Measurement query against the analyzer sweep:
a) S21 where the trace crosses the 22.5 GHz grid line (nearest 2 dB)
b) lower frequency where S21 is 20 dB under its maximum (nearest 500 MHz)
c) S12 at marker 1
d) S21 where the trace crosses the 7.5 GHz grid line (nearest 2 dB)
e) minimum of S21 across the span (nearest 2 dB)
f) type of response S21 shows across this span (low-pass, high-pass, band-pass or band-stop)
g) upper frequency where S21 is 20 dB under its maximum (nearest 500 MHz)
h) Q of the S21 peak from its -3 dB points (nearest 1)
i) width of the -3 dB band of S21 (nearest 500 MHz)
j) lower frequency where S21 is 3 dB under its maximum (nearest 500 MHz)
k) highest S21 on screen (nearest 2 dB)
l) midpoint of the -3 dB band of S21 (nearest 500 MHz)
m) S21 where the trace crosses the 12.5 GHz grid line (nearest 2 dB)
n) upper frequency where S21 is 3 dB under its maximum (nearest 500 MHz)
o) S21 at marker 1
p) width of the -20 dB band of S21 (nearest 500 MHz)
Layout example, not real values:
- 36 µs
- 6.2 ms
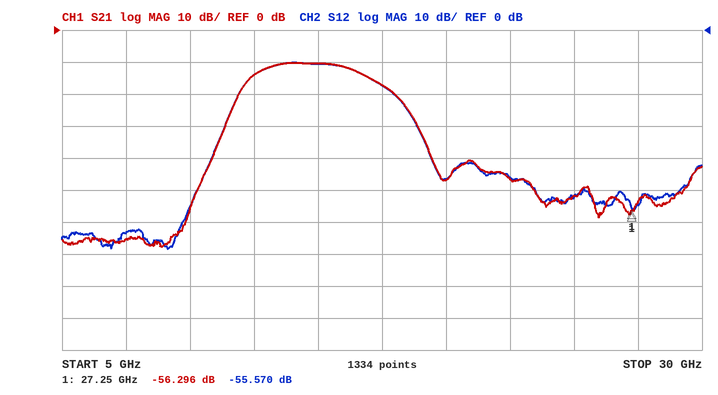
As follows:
- -46 dB
- 11.5 GHz
- -55.570 dB
- -66 dB
- -68 dB
- band-pass
- 19.0 GHz
- 4
- 4.0 GHz
- 12.5 GHz
- -10 dB
- 14.5 GHz
- -14 dB
- 16.5 GHz
- -56.296 dB
- 7.5 GHz
